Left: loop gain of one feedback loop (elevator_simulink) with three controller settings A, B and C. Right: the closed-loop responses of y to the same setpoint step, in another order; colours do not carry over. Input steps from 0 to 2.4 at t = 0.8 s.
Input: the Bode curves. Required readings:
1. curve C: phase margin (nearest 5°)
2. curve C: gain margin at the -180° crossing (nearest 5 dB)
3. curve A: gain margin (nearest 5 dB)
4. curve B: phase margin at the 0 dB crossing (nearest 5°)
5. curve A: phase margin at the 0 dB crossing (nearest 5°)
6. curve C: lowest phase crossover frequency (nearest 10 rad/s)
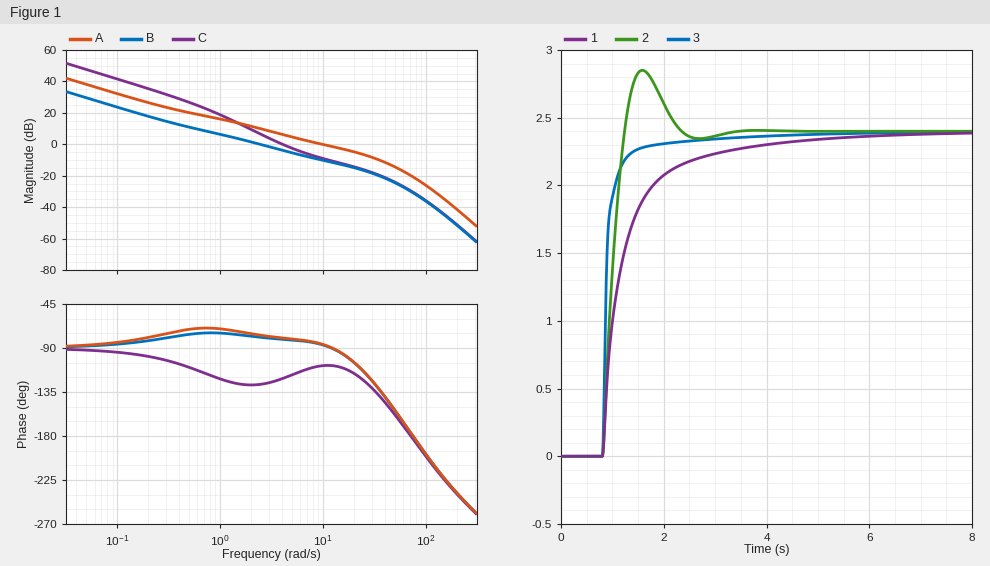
60°
30 dB
20 dB
100°
95°
70 rad/s
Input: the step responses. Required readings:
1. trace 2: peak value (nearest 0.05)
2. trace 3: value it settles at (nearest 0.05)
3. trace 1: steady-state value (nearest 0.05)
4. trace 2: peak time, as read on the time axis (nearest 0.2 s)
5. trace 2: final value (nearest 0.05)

2.85
2.40
2.40
1.6 s
2.40
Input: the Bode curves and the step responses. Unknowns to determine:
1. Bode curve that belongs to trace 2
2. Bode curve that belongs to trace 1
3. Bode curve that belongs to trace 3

C
B
A
